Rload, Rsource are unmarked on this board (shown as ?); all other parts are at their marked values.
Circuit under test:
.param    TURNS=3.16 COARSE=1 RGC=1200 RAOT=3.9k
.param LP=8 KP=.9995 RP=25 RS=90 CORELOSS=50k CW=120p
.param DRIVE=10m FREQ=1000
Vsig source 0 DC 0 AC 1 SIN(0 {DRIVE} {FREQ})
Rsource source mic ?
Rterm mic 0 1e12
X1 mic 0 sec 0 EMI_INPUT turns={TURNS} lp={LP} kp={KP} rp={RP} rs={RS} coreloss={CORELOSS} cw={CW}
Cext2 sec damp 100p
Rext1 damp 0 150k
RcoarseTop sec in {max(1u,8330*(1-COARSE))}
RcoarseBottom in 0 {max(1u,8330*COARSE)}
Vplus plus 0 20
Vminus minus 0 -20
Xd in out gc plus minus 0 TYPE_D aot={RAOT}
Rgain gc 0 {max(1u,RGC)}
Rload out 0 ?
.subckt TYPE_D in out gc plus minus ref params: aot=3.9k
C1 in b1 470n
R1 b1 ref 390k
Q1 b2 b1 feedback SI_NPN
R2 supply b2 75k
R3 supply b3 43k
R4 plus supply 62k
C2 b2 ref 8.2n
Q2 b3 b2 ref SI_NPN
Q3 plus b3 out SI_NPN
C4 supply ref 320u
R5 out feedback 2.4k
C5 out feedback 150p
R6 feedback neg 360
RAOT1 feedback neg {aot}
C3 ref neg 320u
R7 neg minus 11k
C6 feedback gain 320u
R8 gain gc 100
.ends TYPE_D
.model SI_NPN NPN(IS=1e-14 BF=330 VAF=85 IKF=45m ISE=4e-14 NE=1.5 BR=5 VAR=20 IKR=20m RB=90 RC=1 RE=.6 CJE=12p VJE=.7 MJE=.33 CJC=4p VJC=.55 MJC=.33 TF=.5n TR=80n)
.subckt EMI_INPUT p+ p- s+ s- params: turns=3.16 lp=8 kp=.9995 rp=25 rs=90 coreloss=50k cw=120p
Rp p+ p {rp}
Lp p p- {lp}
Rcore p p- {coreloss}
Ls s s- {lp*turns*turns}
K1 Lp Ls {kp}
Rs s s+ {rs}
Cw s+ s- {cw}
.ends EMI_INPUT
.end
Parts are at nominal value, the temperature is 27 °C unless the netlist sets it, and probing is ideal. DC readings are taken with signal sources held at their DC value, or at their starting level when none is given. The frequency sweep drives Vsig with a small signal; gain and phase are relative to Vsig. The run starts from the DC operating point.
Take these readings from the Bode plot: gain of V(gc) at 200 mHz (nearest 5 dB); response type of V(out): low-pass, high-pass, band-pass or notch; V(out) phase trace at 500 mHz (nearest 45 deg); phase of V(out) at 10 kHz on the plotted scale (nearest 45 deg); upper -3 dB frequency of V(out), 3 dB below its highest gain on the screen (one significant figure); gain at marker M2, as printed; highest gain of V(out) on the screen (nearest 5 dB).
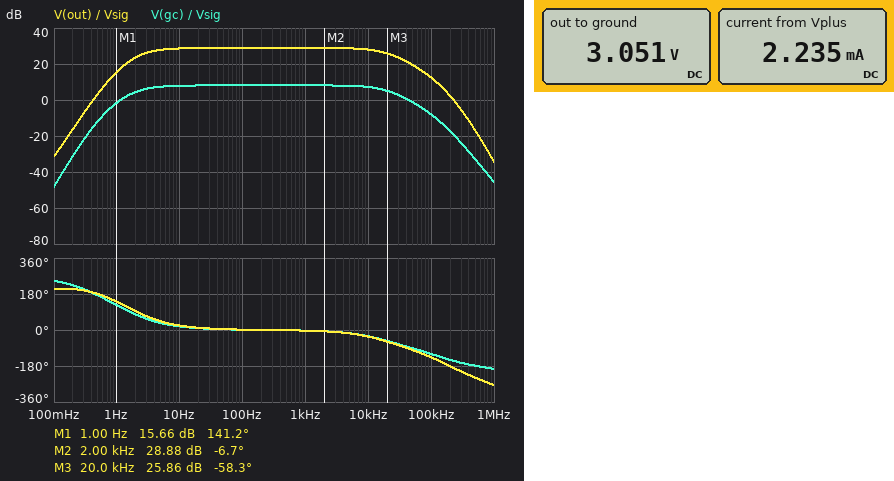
-30 dB
band-pass
180 deg
-45 deg
20 kHz
28.88 dB
30 dB
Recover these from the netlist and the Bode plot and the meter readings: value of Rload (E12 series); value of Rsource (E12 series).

6.8 kΩ
82 Ω
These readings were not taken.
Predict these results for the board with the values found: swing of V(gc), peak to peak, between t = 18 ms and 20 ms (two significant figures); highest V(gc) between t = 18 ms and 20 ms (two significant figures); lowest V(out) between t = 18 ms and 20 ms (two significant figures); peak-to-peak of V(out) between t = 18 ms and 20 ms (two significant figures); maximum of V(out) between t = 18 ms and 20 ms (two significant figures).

51 mV
25 mV
2.8 V
560 mV
3.3 V
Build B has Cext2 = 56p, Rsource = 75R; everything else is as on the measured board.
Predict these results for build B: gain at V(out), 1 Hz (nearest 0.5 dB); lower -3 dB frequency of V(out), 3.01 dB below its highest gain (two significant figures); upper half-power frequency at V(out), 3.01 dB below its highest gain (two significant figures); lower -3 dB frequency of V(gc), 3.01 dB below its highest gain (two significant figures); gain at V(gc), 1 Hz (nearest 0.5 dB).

16.0 dB
2.7 Hz
20 kHz
2.2 Hz
-1.0 dB
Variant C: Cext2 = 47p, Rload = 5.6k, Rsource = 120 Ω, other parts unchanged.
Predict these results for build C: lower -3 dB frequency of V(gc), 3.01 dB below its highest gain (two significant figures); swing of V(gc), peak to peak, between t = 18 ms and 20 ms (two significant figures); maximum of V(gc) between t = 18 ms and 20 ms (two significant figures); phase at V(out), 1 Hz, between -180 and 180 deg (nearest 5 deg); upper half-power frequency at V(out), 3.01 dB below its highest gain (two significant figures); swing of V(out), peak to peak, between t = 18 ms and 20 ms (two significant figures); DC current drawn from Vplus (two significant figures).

2.8 Hz
49 mV
24 mV
145 deg
21 kHz
540 mV
2.3 mA
